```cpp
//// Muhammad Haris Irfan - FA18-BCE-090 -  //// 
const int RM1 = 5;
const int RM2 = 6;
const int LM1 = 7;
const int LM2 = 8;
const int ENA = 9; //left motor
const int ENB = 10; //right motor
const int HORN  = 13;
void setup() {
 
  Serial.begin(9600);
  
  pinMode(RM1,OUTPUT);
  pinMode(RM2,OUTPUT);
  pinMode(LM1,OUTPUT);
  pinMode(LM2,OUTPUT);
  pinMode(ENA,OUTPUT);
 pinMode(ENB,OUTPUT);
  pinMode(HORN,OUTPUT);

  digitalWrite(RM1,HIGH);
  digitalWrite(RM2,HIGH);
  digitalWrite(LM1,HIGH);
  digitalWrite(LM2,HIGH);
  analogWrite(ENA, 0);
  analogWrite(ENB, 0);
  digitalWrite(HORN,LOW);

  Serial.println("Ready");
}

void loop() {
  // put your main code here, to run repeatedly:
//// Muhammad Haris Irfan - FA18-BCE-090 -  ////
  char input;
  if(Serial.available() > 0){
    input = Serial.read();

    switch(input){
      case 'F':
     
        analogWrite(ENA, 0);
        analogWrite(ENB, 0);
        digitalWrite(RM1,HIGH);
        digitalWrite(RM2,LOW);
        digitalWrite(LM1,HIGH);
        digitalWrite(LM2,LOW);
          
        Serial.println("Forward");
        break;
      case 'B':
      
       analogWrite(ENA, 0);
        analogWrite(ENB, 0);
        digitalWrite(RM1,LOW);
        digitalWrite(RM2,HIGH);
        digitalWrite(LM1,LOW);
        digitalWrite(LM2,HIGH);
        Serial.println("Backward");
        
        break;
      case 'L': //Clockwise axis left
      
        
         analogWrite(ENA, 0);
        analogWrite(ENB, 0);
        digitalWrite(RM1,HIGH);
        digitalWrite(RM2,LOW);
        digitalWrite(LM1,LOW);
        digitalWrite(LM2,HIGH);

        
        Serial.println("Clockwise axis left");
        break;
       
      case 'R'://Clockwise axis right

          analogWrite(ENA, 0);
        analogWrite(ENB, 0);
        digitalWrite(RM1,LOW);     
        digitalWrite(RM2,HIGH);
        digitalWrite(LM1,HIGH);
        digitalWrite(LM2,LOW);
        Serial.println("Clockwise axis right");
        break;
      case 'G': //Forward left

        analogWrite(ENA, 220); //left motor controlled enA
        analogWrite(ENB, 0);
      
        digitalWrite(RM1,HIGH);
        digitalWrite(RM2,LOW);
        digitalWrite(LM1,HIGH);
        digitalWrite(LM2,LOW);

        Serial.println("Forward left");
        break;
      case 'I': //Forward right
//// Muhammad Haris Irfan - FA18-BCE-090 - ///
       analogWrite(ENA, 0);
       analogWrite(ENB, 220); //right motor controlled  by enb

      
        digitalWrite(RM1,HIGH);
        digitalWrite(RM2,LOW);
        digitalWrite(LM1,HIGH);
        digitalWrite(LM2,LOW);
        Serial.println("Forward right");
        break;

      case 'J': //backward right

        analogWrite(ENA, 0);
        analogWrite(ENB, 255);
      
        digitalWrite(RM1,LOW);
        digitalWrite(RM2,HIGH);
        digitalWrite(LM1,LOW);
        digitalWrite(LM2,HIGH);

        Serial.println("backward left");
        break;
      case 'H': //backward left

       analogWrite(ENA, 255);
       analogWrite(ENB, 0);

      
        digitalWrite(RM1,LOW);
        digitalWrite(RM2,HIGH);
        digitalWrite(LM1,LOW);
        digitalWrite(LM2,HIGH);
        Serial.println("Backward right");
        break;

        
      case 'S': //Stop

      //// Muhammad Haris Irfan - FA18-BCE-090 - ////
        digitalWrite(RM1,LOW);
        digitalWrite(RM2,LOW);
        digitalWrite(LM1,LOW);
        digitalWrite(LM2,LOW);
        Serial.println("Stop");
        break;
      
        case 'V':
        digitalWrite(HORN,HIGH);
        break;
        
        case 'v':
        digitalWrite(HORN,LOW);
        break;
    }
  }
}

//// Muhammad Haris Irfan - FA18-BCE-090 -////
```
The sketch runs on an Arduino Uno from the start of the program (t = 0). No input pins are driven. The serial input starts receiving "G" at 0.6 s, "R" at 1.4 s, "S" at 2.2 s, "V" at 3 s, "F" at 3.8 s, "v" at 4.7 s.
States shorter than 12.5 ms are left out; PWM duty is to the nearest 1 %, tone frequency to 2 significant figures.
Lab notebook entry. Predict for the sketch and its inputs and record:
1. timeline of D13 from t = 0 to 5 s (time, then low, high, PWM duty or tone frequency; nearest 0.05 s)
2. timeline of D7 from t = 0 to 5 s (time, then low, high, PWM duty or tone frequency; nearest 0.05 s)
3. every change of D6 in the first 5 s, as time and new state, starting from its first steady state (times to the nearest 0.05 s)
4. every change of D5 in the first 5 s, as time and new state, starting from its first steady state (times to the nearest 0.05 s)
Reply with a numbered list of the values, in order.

1. 0 s low; 3 s high; 4.7 s low
2. 0 s high; 2.2 s low; 3.8 s high
3. 0 s high; 0.6 s low; 1.4 s high; 2.2 s low
4. 0 s high; 1.4 s low; 3.8 s high
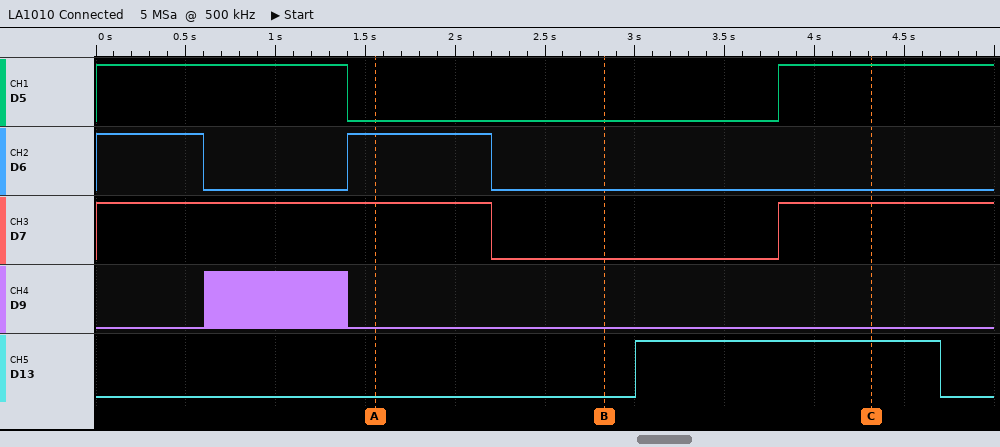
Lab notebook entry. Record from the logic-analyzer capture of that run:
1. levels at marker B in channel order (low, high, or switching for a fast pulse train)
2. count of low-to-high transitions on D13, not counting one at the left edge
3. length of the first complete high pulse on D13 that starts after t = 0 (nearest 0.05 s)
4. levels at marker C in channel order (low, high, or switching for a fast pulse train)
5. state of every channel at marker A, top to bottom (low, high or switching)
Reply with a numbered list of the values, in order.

1. D5 low, D6 low, D7 low, D9 low, D13 low
2. 1
3. 1.70 s
4. D5 high, D6 low, D7 high, D9 low, D13 high
5. D5 low, D6 high, D7 high, D9 low, D13 low
